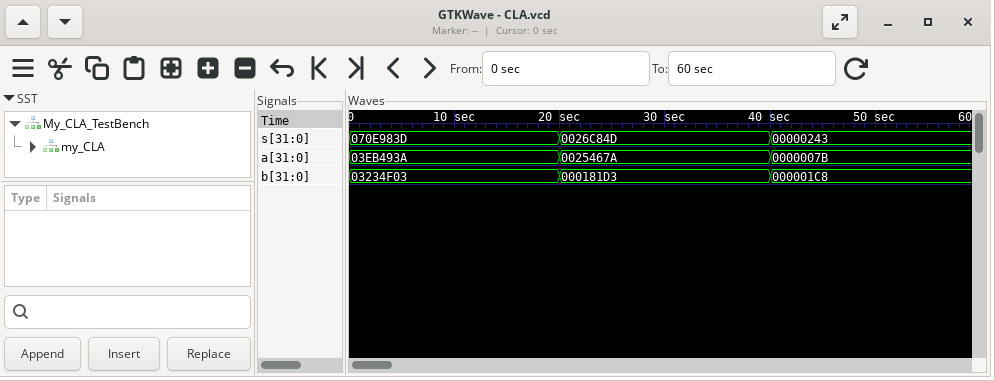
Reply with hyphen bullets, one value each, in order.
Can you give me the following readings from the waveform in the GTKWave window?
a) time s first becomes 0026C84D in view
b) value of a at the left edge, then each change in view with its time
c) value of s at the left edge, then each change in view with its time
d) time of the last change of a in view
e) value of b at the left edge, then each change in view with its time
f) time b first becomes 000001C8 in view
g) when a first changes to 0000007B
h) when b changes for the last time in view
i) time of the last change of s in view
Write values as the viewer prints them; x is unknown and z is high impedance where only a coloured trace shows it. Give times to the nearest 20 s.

- 20 s
- 03EB493A, 0025467A at 20 s, 0000007B at 40 s
- 070E983D, 0026C84D at 20 s, 00000243 at 40 s
- 40 s
- 03234F03, 000181D3 at 20 s, 000001C8 at 40 s
- 40 s
- 40 s
- 40 s
- 40 s
